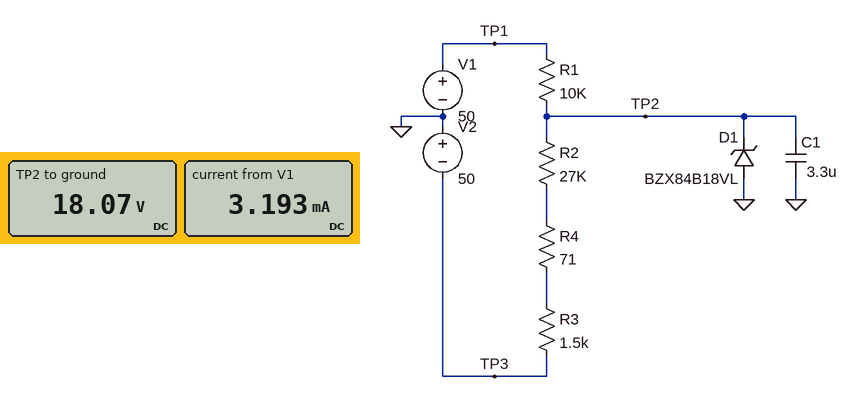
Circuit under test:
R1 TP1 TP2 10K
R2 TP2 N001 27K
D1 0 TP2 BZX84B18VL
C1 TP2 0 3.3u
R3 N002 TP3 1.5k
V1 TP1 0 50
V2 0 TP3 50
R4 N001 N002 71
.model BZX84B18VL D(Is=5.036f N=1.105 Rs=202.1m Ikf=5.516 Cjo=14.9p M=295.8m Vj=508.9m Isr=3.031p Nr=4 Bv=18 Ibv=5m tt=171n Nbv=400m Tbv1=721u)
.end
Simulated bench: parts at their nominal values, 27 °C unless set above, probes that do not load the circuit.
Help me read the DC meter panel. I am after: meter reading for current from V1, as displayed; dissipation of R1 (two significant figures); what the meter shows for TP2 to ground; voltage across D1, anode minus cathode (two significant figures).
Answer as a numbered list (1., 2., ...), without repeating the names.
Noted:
1. 3.193 mA
2. 100 mW
3. 18.07 V
4. -18 V
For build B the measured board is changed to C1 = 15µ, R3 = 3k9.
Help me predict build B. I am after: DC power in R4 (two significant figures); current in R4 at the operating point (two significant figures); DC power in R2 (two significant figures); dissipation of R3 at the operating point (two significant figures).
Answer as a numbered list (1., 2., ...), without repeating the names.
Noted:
1. 340 µW
2. 2.2 mA
3. 130 mW
4. 19 mW
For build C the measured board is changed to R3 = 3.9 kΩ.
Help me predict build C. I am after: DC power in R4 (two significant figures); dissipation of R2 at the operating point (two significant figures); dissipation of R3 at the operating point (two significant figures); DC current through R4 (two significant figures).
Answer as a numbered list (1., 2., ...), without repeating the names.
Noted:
1. 340 µW
2. 130 mW
3. 19 mW
4. 2.2 mA
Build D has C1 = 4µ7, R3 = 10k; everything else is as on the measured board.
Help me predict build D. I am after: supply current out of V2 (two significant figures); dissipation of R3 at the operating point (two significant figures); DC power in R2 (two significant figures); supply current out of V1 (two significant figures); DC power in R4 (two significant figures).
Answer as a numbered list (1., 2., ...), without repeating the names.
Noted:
1. 1.8 mA
2. 34 mW
3. 91 mW
4. 3.2 mA
5. 240 µW
